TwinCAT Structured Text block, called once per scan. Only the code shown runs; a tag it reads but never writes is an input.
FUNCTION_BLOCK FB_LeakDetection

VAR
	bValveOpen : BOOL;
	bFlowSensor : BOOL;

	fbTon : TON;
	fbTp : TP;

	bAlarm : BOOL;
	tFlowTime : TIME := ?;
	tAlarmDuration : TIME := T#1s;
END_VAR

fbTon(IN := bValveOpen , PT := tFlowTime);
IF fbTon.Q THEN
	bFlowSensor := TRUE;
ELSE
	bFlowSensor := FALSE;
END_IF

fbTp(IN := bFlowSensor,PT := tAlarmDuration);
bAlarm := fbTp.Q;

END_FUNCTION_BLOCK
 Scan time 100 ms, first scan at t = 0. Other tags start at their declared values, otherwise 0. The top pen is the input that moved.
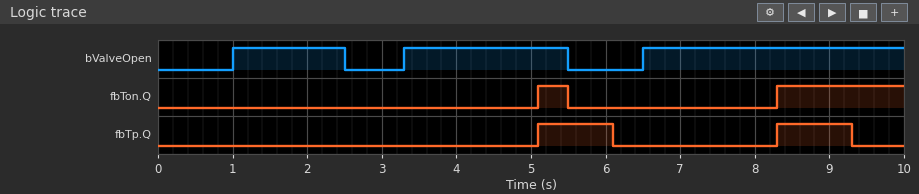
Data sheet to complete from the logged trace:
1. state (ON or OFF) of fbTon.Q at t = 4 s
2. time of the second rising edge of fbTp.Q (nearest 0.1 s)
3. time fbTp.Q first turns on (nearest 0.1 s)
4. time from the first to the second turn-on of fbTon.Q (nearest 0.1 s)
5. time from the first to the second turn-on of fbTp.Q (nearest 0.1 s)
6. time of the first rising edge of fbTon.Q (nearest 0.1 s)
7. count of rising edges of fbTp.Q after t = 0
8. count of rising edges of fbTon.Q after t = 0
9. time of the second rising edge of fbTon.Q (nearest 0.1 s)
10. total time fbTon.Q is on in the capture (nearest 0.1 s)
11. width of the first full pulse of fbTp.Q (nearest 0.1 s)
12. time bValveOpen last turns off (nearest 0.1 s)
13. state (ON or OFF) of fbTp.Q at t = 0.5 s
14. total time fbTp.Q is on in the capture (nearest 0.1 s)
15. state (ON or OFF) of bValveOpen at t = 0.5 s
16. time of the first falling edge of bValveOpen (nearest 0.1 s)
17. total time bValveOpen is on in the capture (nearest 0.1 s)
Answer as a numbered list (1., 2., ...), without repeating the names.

1. OFF
2. 8.3 s
3. 5.1 s
4. 3.2 s
5. 3.2 s
6. 5.1 s
7. 2
8. 2
9. 8.3 s
10. 2.1 s
11. 1.0 s
12. 5.5 s
13. OFF
14. 2.0 s
15. OFF
16. 2.5 s
17. 7.2 s
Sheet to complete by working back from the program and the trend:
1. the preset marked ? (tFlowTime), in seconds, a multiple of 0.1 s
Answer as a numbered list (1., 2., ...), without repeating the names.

1. 1.8 s
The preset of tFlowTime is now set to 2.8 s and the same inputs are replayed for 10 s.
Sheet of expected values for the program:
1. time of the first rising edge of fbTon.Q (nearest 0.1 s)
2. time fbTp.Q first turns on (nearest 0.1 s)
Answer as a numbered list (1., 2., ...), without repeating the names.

1. 9.3 s
2. 9.3 s
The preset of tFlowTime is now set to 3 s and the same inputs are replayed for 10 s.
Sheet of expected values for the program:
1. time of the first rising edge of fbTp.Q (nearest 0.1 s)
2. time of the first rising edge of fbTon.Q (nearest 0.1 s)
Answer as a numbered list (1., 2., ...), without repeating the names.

1. 9.5 s
2. 9.5 s
